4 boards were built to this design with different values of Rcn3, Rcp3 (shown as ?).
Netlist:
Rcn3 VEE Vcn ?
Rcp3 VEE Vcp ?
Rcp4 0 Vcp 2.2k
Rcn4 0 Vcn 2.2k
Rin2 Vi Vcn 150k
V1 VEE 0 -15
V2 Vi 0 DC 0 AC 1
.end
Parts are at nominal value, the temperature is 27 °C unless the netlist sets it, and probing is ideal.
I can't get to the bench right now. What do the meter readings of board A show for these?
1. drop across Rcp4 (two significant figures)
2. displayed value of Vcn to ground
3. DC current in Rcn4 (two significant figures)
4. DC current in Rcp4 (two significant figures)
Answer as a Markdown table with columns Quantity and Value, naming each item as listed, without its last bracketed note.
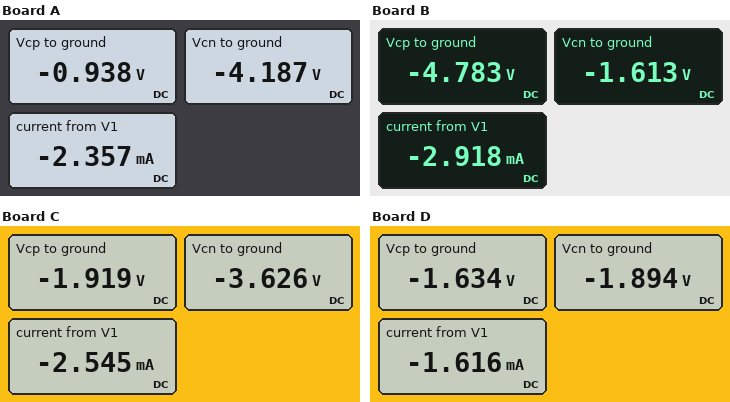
| Quantity | Value |
|---|---|
| drop across Rcp4 | 940 mV |
| displayed value of Vcn to ground | -4.187 V |
| DC current in Rcn4 | 1.9 mA |
| DC current in Rcp4 | 430 µA |
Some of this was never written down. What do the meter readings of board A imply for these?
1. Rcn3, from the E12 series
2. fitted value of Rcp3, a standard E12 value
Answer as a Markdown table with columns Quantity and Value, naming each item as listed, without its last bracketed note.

| Quantity | Value |
|---|---|
| Rcn3, from the E12 series | 5.6 kΩ |
| fitted value of Rcp3, a standard E12 value | 33 kΩ |
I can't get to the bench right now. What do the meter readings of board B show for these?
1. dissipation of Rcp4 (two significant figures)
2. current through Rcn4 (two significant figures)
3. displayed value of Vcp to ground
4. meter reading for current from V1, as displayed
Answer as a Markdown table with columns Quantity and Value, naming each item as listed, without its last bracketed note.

| Quantity | Value |
|---|---|
| dissipation of Rcp4 | 10 mW |
| current through Rcn4 | 730 µA |
| displayed value of Vcp to ground | -4.783 V |
| meter reading for current from V1, as displayed | -2.918 mA |
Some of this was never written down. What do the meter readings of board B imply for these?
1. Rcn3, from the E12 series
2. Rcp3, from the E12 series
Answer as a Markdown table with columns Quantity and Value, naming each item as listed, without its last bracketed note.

| Quantity | Value |
|---|---|
| Rcn3, from the E12 series | 18 kΩ |
| Rcp3, from the E12 series | 4.7 kΩ |
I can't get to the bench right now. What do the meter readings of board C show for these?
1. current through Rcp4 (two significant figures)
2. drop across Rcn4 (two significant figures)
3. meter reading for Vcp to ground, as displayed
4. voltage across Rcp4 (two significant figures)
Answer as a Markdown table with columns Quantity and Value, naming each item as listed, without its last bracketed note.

| Quantity | Value |
|---|---|
| current through Rcp4 | 870 µA |
| drop across Rcn4 | 3.6 V |
| meter reading for Vcp to ground, as displayed | -1.919 V |
| voltage across Rcp4 | 1.9 V |
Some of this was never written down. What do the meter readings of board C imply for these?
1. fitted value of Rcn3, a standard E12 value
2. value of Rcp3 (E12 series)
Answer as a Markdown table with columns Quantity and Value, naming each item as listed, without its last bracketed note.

| Quantity | Value |
|---|---|
| fitted value of Rcn3, a standard E12 value | 6.8 kΩ |
| value of Rcp3 | 15 kΩ |
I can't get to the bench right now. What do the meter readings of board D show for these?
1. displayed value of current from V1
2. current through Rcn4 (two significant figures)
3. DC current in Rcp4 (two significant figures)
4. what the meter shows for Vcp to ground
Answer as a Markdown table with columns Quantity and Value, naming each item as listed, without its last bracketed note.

| Quantity | Value |
|---|---|
| displayed value of current from V1 | -1.616 mA |
| current through Rcn4 | 860 µA |
| DC current in Rcp4 | 740 µA |
| what the meter shows for Vcp to ground | -1.634 V |
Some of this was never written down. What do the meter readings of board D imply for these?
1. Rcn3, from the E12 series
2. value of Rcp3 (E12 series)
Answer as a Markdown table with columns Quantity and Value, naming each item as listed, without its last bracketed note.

| Quantity | Value |
|---|---|
| Rcn3, from the E12 series | 15 kΩ |
| value of Rcp3 | 18 kΩ |
